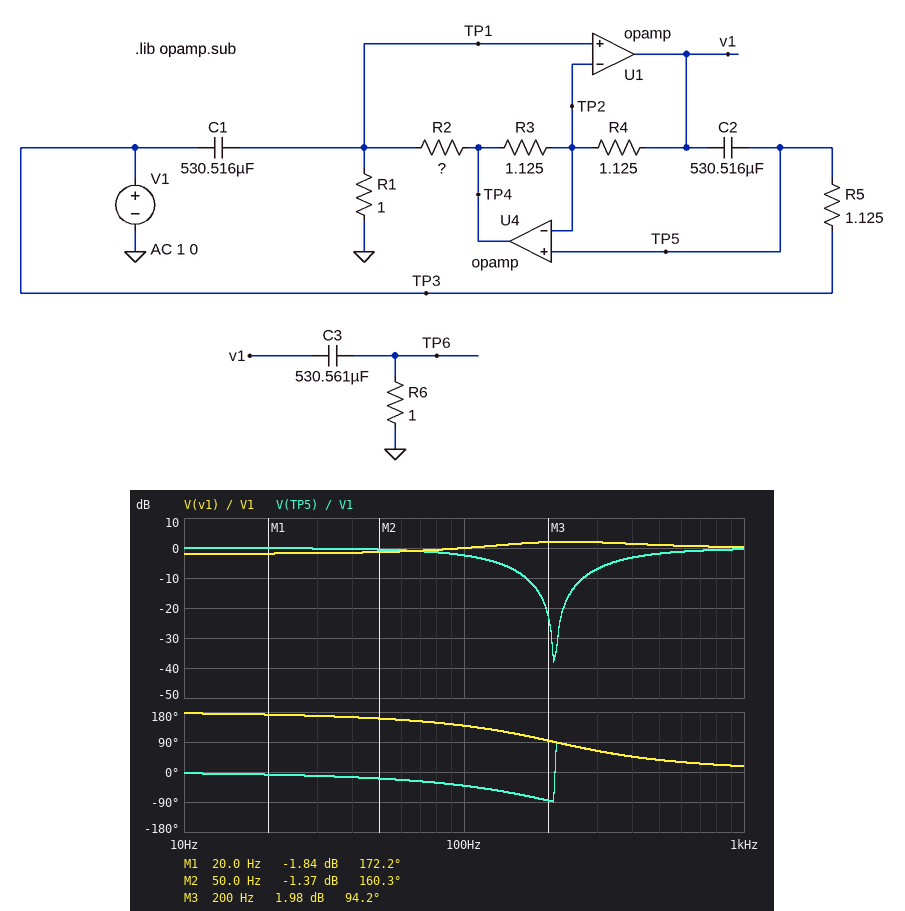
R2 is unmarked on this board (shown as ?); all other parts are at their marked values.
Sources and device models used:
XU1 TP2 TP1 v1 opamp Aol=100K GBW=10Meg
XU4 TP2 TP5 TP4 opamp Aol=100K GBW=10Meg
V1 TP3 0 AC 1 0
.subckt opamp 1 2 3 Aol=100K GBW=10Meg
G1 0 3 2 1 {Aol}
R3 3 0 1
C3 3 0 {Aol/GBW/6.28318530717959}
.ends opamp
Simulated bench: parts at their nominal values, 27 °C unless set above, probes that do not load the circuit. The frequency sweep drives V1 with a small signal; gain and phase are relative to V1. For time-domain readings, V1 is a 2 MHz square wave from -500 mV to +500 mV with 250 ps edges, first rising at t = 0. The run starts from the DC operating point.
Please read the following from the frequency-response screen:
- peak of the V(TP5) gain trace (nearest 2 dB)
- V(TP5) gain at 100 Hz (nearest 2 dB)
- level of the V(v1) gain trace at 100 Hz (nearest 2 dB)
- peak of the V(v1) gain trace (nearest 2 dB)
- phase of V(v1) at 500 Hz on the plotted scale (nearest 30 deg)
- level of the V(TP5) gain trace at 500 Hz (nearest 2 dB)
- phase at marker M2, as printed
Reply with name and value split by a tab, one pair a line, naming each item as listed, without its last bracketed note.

peak of the V(TP5) gain trace	0 dB
V(TP5) gain at 100 Hz	-2 dB
level of the V(v1) gain trace at 100 Hz	0 dB
peak of the V(v1) gain trace	2 dB
phase of V(v1) at 500 Hz on the plotted scale	30 deg
level of the V(TP5) gain trace at 500 Hz	-2 dB
phase at marker M2, as printed	160.3 deg
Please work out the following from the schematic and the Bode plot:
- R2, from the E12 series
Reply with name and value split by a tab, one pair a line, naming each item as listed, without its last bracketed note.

R2, from the E12 series	1.8 Ω
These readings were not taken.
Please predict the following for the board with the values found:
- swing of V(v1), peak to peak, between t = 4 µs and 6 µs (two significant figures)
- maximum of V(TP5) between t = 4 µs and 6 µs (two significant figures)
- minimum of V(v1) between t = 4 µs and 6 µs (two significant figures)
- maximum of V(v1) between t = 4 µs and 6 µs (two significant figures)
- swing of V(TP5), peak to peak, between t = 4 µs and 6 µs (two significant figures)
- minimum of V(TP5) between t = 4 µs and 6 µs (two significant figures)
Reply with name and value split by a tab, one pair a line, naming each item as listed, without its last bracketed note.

swing of V(v1), peak to peak, between t = 4 µs and 6 µs	1.4 V
maximum of V(TP5) between t = 4 µs and 6 µs	700 mV
minimum of V(v1) between t = 4 µs and 6 µs	190 mV
maximum of V(v1) between t = 4 µs and 6 µs	1.6 V
swing of V(TP5), peak to peak, between t = 4 µs and 6 µs	1.4 V
minimum of V(TP5) between t = 4 µs and 6 µs	-710 mV
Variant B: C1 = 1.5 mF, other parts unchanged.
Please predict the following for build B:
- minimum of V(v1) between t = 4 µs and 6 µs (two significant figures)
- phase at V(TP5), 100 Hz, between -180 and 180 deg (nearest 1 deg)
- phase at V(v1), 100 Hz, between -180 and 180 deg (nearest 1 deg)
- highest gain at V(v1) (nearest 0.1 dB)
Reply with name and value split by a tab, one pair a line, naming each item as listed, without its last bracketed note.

minimum of V(v1) between t = 4 µs and 6 µs	190 mV
phase at V(TP5), 100 Hz, between -180 and 180 deg	-62 deg
phase at V(v1), 100 Hz, between -180 and 180 deg	118 deg
highest gain at V(v1)	6.6 dB
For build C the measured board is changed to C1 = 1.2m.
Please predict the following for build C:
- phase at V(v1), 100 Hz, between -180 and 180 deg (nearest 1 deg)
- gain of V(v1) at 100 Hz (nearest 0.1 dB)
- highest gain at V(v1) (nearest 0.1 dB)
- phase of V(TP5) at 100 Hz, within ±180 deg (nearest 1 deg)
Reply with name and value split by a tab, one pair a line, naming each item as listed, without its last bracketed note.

phase at V(v1), 100 Hz, between -180 and 180 deg	126 deg
gain of V(v1) at 100 Hz	3.9 dB
highest gain at V(v1)	5.6 dB
phase of V(TP5) at 100 Hz, within ±180 deg	-54 deg
